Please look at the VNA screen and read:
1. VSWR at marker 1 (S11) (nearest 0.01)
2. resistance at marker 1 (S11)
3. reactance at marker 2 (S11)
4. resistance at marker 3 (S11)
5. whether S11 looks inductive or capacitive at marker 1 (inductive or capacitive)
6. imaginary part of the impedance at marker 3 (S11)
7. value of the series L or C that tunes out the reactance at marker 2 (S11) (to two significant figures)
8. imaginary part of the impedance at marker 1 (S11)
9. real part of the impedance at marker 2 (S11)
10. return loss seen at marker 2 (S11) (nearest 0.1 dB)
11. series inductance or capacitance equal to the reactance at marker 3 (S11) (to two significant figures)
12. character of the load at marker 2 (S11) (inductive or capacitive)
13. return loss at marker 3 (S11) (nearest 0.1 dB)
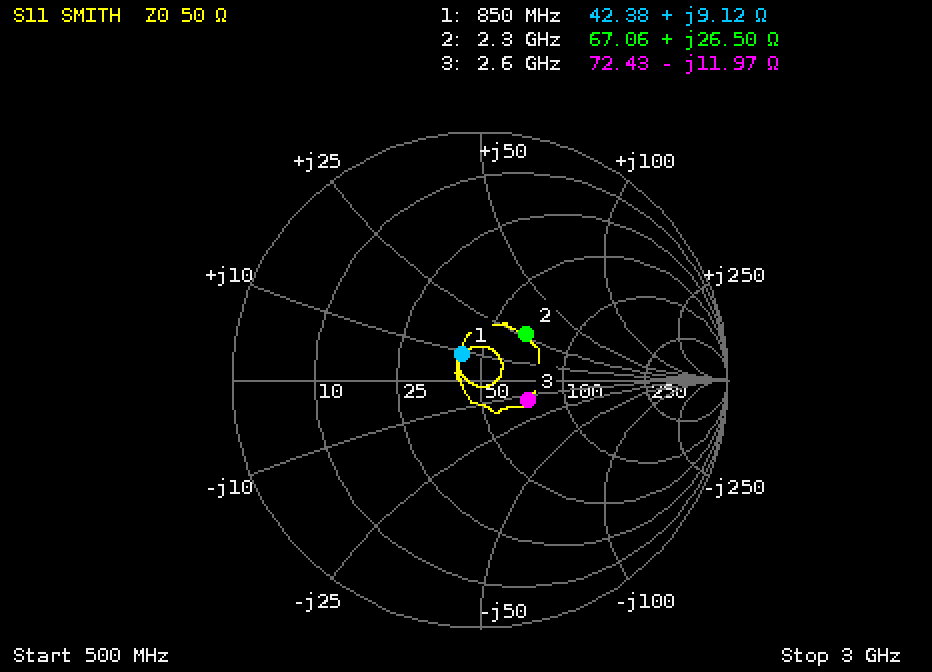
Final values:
1.29
42.38 Ω
+26.50 Ω
72.43 Ω
inductive
-11.97 Ω
2.6 pF
+9.12 Ω
67.06 Ω
11.6 dB
5.1 pF
inductive
13.7 dB
